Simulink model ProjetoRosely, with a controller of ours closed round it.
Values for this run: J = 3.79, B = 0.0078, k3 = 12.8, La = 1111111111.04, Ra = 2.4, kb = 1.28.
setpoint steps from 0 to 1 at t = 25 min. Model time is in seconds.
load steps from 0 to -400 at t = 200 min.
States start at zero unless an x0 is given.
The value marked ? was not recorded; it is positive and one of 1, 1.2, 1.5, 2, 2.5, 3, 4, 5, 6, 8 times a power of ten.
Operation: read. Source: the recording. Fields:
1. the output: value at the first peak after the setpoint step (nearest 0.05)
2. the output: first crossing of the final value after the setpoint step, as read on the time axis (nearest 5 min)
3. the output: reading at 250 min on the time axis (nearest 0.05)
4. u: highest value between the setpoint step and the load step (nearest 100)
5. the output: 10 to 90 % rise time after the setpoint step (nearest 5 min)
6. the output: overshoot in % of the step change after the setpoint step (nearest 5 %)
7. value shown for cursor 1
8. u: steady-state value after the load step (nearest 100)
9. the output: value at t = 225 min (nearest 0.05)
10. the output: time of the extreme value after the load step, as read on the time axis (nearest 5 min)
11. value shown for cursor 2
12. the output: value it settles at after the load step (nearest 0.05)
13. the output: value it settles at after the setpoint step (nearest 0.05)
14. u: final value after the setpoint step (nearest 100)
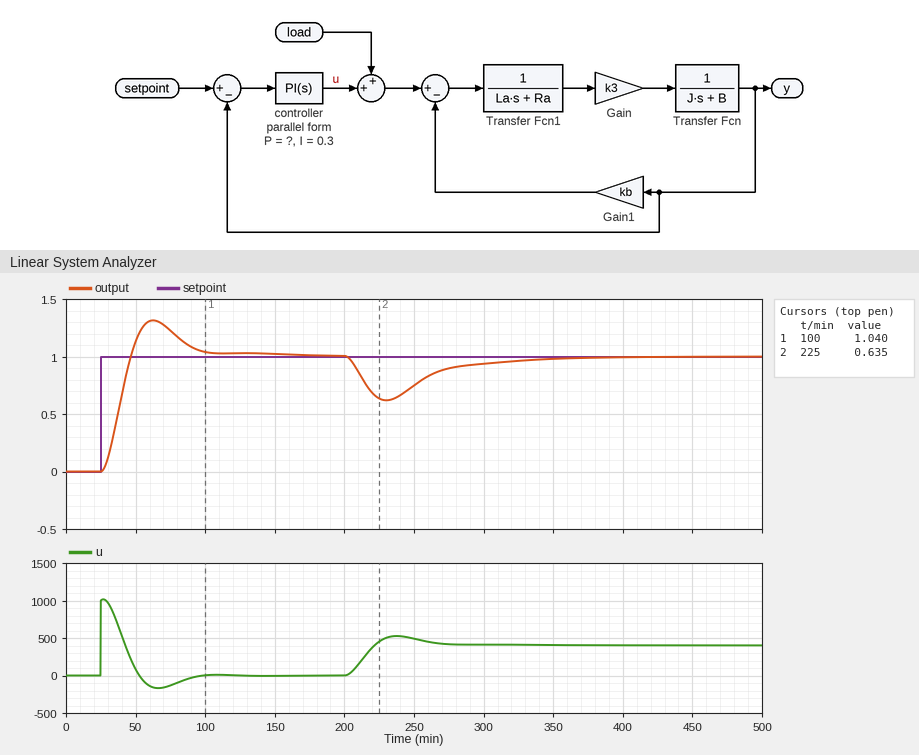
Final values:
1.30
45 min
0.75
1000
15 min
30 %
1.040
400
0.65
230 min
0.635
1.00
1.00
0
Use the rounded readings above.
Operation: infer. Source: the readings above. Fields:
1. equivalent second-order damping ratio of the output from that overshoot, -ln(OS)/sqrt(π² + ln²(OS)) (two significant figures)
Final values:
0.36
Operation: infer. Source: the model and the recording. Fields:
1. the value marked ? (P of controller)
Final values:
1000
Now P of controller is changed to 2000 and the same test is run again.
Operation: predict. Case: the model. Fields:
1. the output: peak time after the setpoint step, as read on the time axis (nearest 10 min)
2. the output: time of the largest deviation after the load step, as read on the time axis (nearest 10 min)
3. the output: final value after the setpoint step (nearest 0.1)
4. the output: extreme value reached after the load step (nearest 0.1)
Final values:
50 min
220 min
1.0
0.8
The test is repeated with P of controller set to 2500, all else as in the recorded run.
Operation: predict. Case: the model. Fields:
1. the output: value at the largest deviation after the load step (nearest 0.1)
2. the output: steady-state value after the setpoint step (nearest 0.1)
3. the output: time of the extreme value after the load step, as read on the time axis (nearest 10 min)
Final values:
0.8
1.0
220 min
